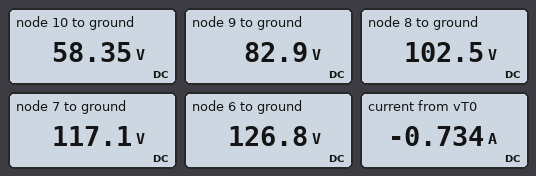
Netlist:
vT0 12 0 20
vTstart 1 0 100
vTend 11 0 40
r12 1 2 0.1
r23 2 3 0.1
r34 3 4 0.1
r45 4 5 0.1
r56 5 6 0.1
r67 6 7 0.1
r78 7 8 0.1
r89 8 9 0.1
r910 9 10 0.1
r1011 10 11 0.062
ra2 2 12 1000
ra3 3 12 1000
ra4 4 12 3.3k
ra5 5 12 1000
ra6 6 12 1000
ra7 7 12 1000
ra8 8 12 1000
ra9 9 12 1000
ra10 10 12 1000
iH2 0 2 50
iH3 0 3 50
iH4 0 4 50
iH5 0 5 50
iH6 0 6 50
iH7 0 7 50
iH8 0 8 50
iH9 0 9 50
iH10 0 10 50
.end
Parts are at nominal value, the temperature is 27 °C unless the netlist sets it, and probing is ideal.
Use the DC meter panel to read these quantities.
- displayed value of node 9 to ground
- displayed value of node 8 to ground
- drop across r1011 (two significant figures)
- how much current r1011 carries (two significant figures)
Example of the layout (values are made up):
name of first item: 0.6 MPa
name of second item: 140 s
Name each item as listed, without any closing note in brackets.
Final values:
displayed value of node 9 to ground: 82.9 V
displayed value of node 8 to ground: 102.5 V
drop across r1011: 18 V
how much current r1011 carries: 300 A
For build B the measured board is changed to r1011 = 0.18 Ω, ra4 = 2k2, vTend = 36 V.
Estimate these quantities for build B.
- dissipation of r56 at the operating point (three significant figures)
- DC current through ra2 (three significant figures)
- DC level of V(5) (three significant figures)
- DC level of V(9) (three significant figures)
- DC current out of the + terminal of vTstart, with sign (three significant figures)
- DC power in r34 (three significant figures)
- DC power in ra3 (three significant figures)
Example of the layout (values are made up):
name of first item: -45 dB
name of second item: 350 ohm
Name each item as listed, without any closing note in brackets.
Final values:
dissipation of r56 at the operating point: 31.3 W
DC current through ra2: 98.2 mA
DC level of V(5): 143 V
DC level of V(9): 106 V
DC current out of the + terminal of vTstart, with sign: -182 A
DC power in r34: 675 W
DC power in ra3: 12.4 W
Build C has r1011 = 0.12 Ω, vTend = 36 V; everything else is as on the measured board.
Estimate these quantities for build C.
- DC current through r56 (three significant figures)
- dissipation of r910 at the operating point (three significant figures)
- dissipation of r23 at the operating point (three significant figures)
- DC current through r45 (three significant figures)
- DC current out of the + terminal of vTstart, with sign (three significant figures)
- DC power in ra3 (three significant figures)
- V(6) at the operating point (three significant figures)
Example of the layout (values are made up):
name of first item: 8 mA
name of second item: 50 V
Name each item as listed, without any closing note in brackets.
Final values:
DC current through r56: 33.4 A
dissipation of r910 at the operating point: 5.43 kW
dissipation of r23 at the operating point: 1.35 kW
DC current through r45: 16.5 A
DC current out of the + terminal of vTstart, with sign: -166 A
DC power in ra3: 11.7 W
V(6) at the operating point: 133 V
